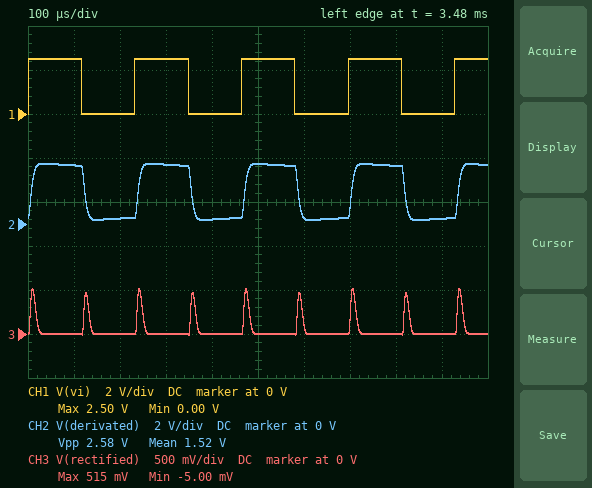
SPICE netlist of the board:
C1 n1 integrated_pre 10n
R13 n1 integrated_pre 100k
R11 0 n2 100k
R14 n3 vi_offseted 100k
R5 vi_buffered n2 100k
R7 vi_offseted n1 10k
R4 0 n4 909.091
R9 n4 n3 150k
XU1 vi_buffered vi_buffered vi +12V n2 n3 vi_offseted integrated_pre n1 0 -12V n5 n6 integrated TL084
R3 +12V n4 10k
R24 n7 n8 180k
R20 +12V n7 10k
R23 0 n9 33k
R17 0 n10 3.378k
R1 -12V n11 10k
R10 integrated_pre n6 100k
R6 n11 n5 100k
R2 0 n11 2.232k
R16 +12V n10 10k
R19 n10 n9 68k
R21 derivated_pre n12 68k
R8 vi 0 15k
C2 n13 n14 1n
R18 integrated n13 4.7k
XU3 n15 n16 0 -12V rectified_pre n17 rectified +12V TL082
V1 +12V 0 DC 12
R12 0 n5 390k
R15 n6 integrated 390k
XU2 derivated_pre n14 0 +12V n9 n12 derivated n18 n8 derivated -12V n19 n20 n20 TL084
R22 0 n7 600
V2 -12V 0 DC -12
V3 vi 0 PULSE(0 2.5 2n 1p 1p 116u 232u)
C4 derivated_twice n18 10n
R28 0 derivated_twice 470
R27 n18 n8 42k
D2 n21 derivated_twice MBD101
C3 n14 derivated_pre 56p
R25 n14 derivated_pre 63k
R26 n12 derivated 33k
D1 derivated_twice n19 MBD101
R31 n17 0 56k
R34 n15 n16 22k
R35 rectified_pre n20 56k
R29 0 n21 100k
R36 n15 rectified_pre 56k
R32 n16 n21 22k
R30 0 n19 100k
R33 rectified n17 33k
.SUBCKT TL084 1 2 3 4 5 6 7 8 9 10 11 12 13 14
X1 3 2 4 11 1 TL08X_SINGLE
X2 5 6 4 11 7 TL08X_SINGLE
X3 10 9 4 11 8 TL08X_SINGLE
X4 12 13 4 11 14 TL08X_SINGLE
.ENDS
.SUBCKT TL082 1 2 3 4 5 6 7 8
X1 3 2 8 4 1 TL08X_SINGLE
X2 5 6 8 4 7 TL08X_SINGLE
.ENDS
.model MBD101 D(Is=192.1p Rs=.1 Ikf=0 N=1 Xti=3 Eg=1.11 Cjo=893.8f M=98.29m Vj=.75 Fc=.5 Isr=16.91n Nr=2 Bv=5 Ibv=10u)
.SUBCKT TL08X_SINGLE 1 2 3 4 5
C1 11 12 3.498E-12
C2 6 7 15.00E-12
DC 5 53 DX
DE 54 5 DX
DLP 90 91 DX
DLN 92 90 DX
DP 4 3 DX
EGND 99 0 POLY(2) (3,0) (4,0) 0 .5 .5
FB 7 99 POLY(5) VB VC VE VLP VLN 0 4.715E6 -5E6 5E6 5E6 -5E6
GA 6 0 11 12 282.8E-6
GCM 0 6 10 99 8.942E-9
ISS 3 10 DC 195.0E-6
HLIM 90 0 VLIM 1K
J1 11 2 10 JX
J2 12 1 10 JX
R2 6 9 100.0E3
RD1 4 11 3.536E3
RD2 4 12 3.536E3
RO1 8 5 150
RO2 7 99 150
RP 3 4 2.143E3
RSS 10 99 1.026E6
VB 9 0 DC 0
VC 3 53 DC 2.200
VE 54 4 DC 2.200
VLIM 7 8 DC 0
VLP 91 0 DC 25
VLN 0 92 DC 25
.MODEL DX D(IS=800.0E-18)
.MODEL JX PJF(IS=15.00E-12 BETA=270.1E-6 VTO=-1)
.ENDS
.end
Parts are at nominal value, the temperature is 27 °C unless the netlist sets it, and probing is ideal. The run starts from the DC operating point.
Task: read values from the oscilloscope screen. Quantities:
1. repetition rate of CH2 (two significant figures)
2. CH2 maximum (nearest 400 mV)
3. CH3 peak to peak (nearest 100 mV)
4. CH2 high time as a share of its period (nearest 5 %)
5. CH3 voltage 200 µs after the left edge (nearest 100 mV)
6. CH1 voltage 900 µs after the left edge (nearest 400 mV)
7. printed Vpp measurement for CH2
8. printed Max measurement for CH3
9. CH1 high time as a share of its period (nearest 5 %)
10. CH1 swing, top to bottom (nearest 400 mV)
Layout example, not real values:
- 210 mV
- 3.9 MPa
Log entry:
- 4.3 kHz
- 2.8 V
- 500 mV
- 50 %
- 0 V
- 0 V
- 2.58 V
- 515 mV
- 50 %
- 2.4 V
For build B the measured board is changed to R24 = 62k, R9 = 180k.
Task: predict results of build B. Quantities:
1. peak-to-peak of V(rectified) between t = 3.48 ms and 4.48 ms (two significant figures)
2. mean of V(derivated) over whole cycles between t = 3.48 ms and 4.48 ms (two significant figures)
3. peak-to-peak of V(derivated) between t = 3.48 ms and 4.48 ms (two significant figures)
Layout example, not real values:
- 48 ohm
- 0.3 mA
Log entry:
- 710 mV
- 1.5 V
- 2.4 V
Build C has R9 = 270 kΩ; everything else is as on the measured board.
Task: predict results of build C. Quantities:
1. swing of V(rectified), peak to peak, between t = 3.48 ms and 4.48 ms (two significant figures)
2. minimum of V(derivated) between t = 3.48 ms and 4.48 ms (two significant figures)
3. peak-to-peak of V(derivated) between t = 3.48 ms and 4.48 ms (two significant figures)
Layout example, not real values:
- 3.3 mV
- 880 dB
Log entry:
- 400 mV
- 440 mV
- 2.1 V
